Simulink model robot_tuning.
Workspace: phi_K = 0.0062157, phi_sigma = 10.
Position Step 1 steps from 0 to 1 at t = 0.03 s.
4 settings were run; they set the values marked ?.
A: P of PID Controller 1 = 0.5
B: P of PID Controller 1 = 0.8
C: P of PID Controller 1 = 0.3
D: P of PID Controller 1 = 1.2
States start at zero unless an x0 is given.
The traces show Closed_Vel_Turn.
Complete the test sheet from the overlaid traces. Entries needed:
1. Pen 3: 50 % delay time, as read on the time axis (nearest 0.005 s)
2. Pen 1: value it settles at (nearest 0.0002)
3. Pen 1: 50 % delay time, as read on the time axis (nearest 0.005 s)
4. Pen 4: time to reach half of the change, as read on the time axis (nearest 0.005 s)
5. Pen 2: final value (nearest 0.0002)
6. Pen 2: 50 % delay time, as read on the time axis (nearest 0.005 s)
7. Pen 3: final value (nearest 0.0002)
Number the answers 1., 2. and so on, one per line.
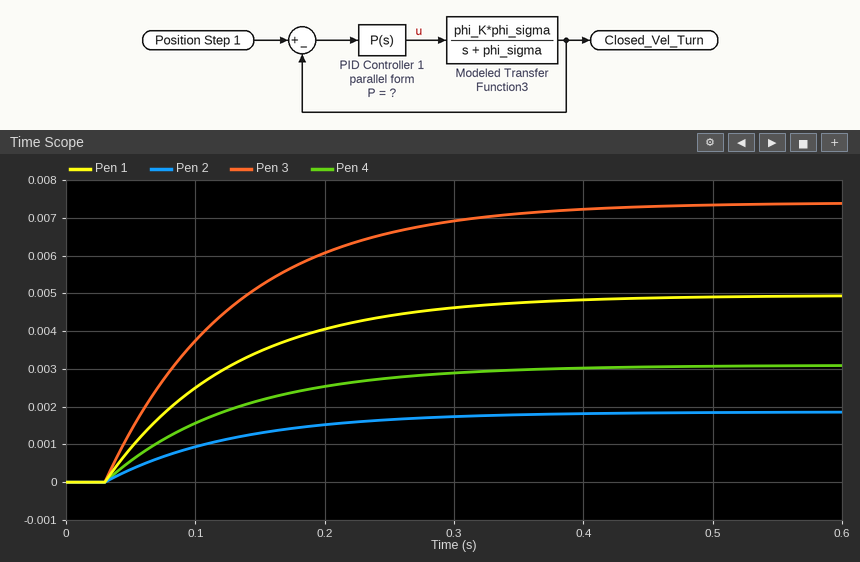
1. 0.100 s
2. 0.0050
3. 0.100 s
4. 0.100 s
5. 0.0018
6. 0.100 s
7. 0.0074
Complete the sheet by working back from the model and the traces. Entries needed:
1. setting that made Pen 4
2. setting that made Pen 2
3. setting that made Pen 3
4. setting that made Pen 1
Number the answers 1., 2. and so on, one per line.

1. A
2. C
3. D
4. B
